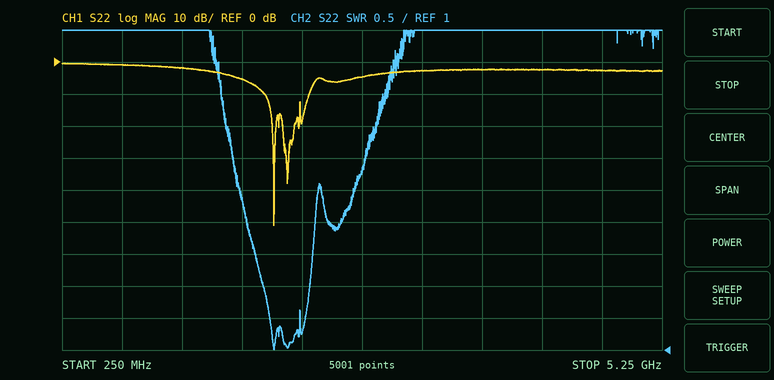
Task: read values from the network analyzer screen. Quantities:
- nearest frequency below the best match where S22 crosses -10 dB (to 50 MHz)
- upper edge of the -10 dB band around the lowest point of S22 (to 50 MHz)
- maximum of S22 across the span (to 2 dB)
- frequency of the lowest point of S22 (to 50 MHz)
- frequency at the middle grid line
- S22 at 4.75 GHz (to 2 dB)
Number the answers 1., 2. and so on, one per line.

1. 1.95 GHz
2. 2.30 GHz
3. 0 dB
4. 2.00 GHz
5. 2.75 GHz
6. -2 dB
